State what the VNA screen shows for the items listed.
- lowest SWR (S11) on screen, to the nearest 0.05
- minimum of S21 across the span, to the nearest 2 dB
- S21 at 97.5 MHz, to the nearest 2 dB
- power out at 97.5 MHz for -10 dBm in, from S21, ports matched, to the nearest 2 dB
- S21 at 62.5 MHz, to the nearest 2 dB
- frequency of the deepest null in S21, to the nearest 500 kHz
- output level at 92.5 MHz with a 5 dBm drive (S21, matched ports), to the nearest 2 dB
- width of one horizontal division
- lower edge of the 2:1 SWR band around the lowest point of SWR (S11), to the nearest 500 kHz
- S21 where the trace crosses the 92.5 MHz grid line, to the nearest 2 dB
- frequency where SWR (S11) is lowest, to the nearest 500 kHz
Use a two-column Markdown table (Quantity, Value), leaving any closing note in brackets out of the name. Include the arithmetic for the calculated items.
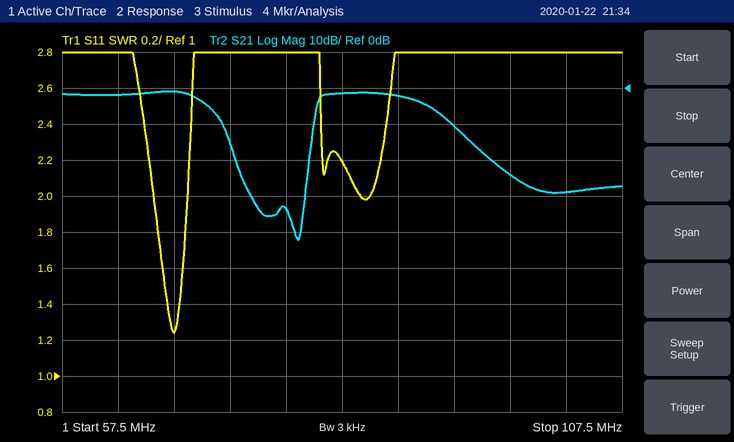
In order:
| Quantity | Value |
|---|---|
| lowest SWR (S11) on screen, to the nearest 0.05 | 1.25 |
| minimum of S21 across the span, to the nearest 2 dB | -42 dB |
| S21 at 97.5 MHz, to the nearest 2 dB | -24 dB |
| power out at 97.5 MHz for -10 dBm in, from S21, ports matched, to the nearest 2 dB | -10 dBm + (-24 dB) = -34 dBm |
| S21 at 62.5 MHz, to the nearest 2 dB | -2 dB |
| frequency of the deepest null in S21, to the nearest 500 kHz | 78.5 MHz |
| output level at 92.5 MHz with a 5 dBm drive (S21, matched ports), to the nearest 2 dB | 5 dBm + (-10 dB) = -6 dBm |
| width of one horizontal division | 5 MHz |
| lower edge of the 2:1 SWR band around the lowest point of SWR (S11), to the nearest 500 kHz | 65.5 MHz |
| S21 where the trace crosses the 92.5 MHz grid line, to the nearest 2 dB | -10 dB |
| frequency where SWR (S11) is lowest, to the nearest 500 kHz | 67.5 MHz |
